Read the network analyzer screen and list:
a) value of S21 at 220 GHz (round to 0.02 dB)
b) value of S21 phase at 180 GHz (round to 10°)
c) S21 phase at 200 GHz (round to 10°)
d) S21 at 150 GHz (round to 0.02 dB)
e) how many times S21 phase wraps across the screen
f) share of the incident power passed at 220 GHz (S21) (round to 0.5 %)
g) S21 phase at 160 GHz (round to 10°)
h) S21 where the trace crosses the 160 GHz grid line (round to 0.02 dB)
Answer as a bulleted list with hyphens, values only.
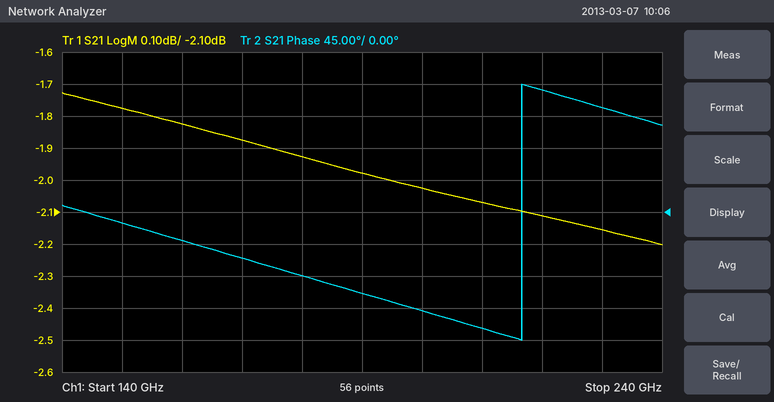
- -2.12 dB
- -90°
- -140°
- -1.78 dB
- 1
- 61.5 %
- -40°
- -1.82 dB
